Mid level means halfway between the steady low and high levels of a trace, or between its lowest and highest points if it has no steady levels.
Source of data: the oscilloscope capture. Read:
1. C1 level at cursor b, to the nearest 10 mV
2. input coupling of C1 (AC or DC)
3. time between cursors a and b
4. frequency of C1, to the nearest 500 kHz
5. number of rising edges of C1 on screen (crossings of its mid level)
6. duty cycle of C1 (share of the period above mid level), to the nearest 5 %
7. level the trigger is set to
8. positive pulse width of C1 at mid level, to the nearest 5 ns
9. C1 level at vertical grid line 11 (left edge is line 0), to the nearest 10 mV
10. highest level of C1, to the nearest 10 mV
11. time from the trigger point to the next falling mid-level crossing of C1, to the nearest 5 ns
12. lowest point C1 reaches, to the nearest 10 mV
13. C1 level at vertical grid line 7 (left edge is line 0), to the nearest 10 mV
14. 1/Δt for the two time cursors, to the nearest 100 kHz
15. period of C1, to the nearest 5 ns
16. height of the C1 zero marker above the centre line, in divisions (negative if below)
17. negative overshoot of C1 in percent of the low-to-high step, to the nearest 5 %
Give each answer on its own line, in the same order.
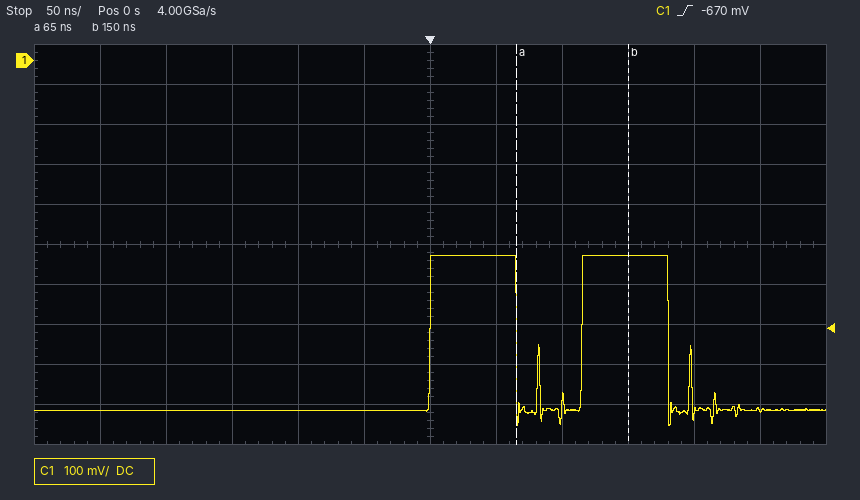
-490 mV
DC
85 ns
8.5 MHz
2
55 %
-670 mV
65 ns
-870 mV
-490 mV
65 ns
-910 mV
-490 mV
11.8 MHz
115 ns
+4.6 div
10 %
